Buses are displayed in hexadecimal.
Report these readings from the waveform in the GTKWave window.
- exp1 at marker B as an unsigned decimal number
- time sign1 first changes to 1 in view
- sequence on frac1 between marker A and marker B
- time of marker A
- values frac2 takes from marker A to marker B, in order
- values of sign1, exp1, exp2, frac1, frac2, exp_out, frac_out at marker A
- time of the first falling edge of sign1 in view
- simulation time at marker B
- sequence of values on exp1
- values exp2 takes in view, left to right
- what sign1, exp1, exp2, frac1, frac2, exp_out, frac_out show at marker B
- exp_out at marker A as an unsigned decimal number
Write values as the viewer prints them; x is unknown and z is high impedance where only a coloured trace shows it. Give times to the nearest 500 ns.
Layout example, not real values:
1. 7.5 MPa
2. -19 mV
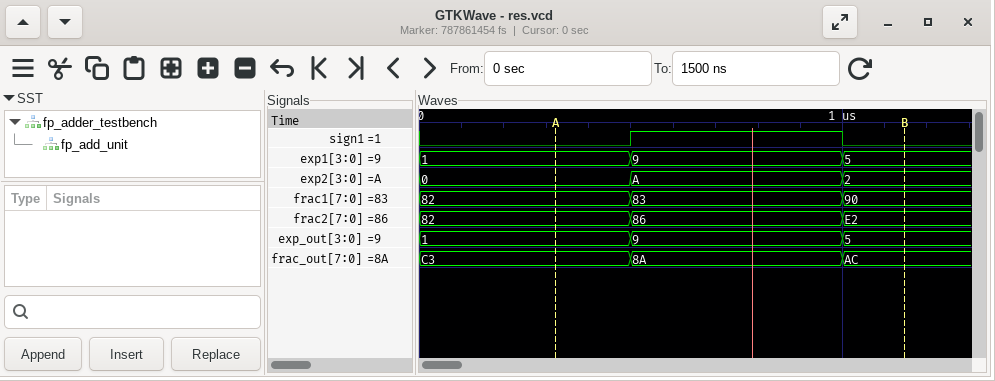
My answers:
1. 5
2. 500 ns
3. 82, 83, 90
4. 500 ns
5. 82, 86, E2
6. sign1=0, exp1=1, exp2=0, frac1=82, frac2=82, exp_out=1, frac_out=C3
7. 1000 ns
8. 1000 ns
9. 1, 9, 5
10. 0, A, 2
11. sign1=0, exp1=5, exp2=2, frac1=90, frac2=E2, exp_out=5, frac_out=AC
12. 1
